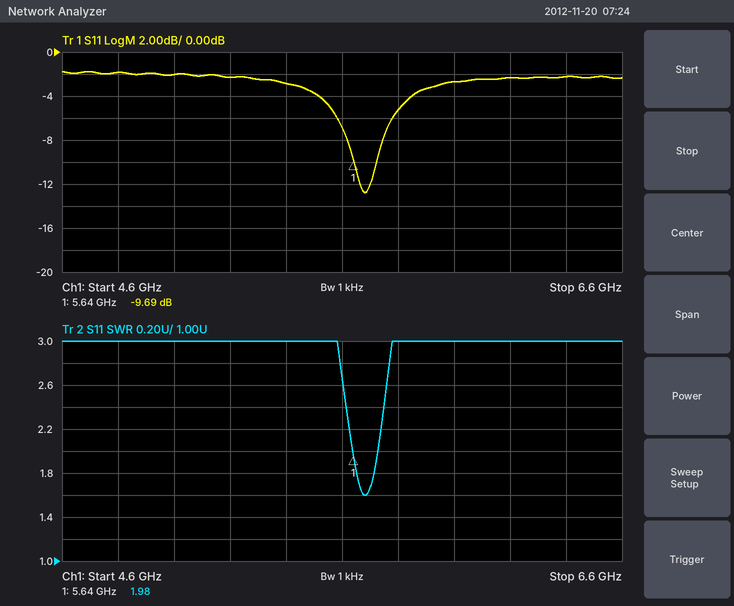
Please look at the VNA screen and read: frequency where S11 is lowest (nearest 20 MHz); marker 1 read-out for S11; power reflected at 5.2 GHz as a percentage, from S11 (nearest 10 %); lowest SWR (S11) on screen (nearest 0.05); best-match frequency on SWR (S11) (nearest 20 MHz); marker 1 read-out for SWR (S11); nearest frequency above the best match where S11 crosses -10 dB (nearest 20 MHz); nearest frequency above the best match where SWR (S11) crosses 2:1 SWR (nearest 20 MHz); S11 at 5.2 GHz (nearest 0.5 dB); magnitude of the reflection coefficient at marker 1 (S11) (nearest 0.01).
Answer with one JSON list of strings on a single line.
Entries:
["5.68 GHz", "-9.69 dB", "60 %", "1.60", "5.68 GHz", "1.98", "5.72 GHz", "5.72 GHz", "-2.5 dB", "0.33"]
